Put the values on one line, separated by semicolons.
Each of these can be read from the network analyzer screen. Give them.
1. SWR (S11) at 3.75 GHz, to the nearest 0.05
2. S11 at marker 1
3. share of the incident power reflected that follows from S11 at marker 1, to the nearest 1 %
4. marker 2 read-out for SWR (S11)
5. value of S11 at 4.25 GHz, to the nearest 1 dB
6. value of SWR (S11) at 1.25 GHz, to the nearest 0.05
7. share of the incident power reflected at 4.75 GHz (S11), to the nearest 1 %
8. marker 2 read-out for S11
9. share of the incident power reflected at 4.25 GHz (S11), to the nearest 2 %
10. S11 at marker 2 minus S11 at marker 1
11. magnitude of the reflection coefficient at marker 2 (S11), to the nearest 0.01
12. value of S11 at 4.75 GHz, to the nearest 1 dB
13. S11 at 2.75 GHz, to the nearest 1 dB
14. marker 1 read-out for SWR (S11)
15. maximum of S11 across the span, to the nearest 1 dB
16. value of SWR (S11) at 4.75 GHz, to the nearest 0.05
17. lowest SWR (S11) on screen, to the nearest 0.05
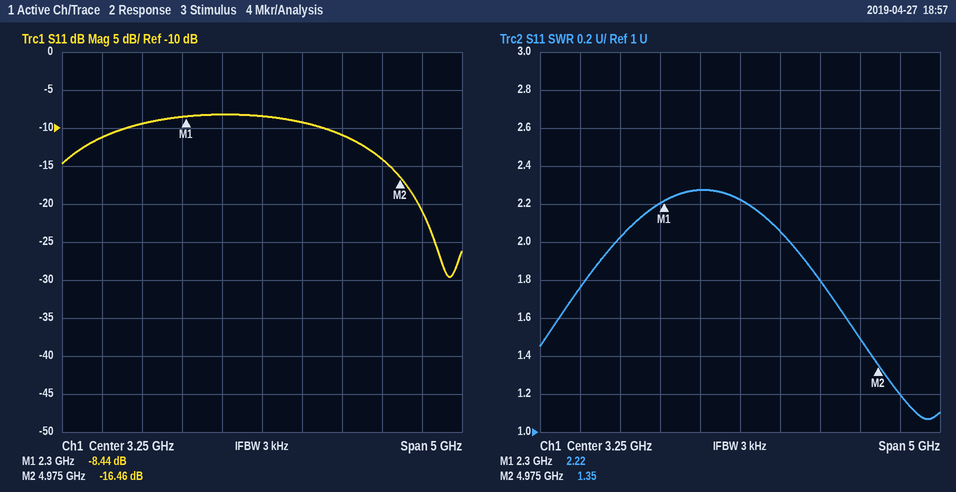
2.05; -8.44 dB; 14 %; 1.35; -11 dB; 1.75; 4 %; -16.46 dB; 8 %; -8.02 dB; 0.15; -14 dB; -8 dB; 2.22; -8 dB; 1.50; 1.05
